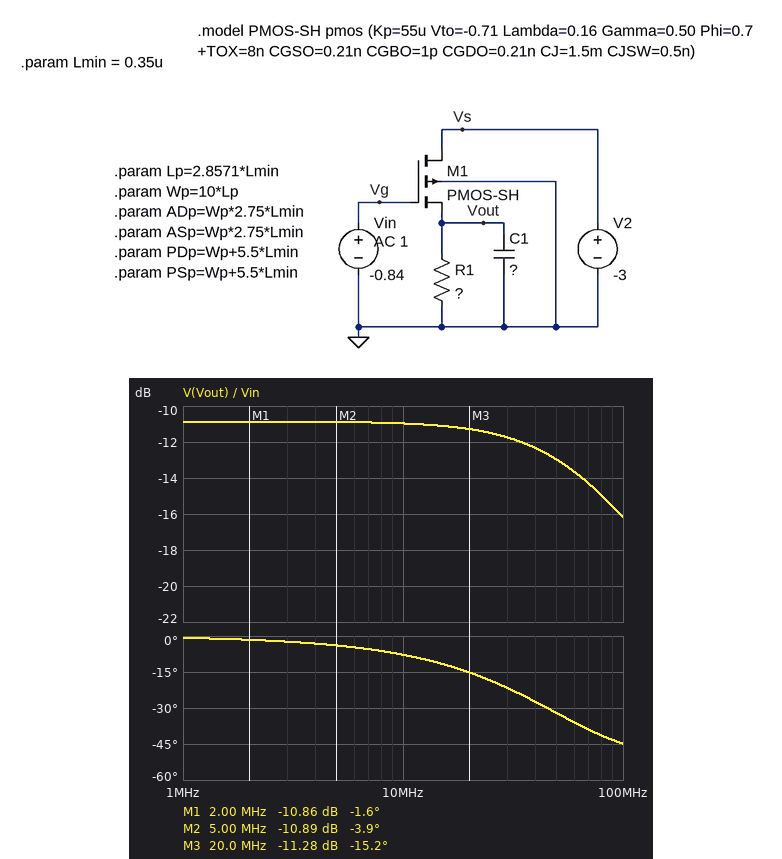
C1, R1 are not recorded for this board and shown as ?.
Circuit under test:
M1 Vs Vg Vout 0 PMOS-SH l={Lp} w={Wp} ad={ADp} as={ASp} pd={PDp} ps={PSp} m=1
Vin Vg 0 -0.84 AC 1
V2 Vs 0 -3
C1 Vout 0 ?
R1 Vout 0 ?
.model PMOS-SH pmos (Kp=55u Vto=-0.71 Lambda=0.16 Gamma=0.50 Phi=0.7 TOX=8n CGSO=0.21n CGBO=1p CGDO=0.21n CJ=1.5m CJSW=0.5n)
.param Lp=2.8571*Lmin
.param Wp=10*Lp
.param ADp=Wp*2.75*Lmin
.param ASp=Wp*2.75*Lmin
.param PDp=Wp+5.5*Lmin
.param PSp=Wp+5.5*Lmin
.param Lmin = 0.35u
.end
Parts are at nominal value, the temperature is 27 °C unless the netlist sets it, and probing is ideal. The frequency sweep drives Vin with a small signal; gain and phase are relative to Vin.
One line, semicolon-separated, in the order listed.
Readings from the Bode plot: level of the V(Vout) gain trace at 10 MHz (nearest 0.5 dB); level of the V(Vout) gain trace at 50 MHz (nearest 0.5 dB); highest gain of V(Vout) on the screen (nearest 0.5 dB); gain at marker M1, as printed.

-11.0 dB; -13.0 dB; -11.0 dB; -10.86 dB
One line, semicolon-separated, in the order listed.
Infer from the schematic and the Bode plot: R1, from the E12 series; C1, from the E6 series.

5.6 kΩ; 680 fF
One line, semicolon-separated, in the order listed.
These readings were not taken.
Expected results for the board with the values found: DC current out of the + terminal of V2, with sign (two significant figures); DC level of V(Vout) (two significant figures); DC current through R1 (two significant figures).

-4.1 µA; -23 mV; 4.1 µA
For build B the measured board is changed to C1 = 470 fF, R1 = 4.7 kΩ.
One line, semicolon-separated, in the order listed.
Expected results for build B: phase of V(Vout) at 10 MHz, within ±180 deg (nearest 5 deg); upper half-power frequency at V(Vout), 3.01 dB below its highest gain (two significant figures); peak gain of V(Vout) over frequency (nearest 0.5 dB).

-5 deg; 100 MHz; -11.5 dB
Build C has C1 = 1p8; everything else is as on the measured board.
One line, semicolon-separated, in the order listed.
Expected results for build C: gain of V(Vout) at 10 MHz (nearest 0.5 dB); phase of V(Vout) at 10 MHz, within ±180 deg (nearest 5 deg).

-11.5 dB; -20 deg
